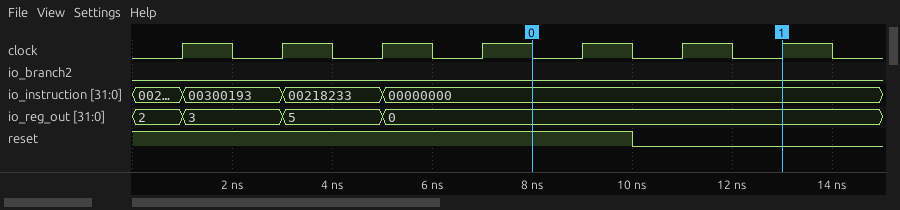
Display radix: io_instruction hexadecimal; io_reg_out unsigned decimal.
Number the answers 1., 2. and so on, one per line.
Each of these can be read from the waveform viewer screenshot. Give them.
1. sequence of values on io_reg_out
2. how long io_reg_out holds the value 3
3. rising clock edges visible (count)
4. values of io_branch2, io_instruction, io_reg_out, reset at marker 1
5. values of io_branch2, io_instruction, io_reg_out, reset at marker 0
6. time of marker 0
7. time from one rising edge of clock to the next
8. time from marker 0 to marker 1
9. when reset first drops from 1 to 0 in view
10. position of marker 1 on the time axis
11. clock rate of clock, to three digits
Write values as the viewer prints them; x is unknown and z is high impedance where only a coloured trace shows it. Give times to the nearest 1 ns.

1. 2, 3, 5, 0
2. 2 ns
3. 7
4. io_branch2=0, io_instruction=00000000, io_reg_out=0, reset=0
5. io_branch2=0, io_instruction=00000000, io_reg_out=0, reset=1
6. 8 ns
7. 2 ns
8. 5 ns
9. 10 ns
10. 13 ns
11. 500 MHz
